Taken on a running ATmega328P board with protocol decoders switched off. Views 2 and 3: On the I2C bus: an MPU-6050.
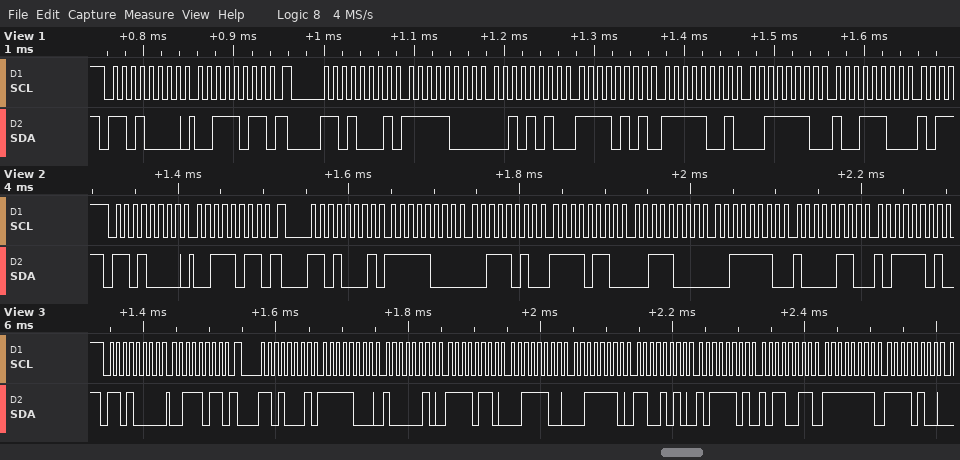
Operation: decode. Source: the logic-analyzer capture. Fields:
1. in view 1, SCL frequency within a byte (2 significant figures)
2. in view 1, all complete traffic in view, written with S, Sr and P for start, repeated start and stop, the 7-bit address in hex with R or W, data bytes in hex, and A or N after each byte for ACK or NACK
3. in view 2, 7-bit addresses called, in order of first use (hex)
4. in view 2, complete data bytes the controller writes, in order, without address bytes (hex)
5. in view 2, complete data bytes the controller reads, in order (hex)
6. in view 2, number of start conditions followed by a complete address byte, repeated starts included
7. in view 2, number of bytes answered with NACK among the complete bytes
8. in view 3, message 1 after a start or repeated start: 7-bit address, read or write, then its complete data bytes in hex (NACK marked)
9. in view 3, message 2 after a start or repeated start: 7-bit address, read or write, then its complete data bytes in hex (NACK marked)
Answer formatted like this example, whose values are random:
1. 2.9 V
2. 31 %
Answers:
1. 100 kHz
2. S 68W A 3B A Sr 68R A F8 A 2A A F5 A F9 A 3E A 9C A
3. 0x68
4. 3B
5. F8 3A F6 38 3E 86 BD
6. 2
7. 0
8. 0x68 write: 3B
9. 0x68 read: F8 82 F6 3C 3E CA BD B3 FF F4
